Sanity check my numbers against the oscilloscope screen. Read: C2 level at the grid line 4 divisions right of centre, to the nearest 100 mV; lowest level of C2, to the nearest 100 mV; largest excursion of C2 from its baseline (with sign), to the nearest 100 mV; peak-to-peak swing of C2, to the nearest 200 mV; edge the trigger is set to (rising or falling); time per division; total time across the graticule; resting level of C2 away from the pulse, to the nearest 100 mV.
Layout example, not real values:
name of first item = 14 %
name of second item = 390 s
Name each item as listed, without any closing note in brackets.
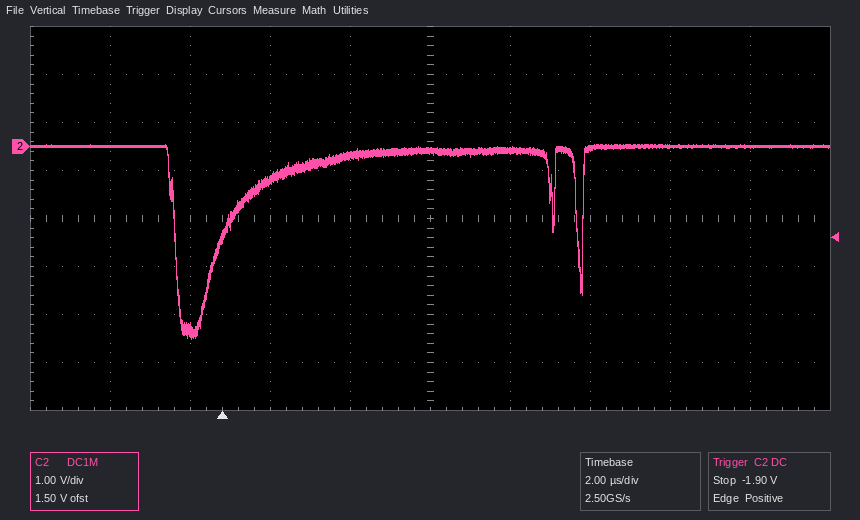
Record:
C2 level at the grid line 4 divisions right of centre, to the nearest 100 mV = 0.0 V
lowest level of C2, to the nearest 100 mV = -4.0 V
largest excursion of C2 from its baseline (with sign), to the nearest 100 mV = -4.0 V
peak-to-peak swing of C2, to the nearest 200 mV = 4.0 V
edge the trigger is set to = rising
time per division = 2 µs
total time across the graticule = 20 µs
resting level of C2 away from the pulse, to the nearest 100 mV = 0.0 V
